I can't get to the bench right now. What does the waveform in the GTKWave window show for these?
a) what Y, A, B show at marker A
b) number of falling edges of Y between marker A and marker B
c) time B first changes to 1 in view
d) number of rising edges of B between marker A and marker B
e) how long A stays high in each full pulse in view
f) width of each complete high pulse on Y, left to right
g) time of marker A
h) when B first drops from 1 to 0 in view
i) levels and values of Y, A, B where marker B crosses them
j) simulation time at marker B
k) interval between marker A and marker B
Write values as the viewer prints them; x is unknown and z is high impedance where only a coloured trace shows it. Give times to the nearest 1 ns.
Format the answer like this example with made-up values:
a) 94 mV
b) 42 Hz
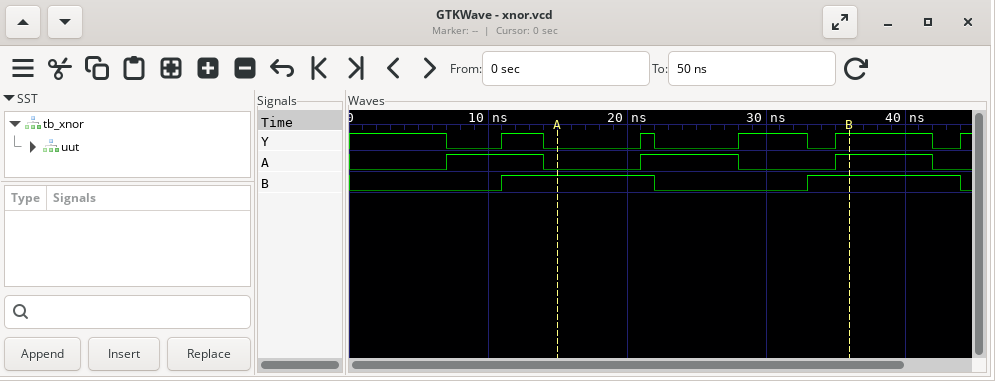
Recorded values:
a) Y=0, A=0, B=1
b) 2
c) 11 ns
d) 1
e) 7 ns, 7 ns, 7 ns
f) 3 ns, 1 ns, 5 ns, 7 ns
g) 15 ns
h) 22 ns
i) Y=1, A=1, B=1
j) 36 ns
k) 21 ns
